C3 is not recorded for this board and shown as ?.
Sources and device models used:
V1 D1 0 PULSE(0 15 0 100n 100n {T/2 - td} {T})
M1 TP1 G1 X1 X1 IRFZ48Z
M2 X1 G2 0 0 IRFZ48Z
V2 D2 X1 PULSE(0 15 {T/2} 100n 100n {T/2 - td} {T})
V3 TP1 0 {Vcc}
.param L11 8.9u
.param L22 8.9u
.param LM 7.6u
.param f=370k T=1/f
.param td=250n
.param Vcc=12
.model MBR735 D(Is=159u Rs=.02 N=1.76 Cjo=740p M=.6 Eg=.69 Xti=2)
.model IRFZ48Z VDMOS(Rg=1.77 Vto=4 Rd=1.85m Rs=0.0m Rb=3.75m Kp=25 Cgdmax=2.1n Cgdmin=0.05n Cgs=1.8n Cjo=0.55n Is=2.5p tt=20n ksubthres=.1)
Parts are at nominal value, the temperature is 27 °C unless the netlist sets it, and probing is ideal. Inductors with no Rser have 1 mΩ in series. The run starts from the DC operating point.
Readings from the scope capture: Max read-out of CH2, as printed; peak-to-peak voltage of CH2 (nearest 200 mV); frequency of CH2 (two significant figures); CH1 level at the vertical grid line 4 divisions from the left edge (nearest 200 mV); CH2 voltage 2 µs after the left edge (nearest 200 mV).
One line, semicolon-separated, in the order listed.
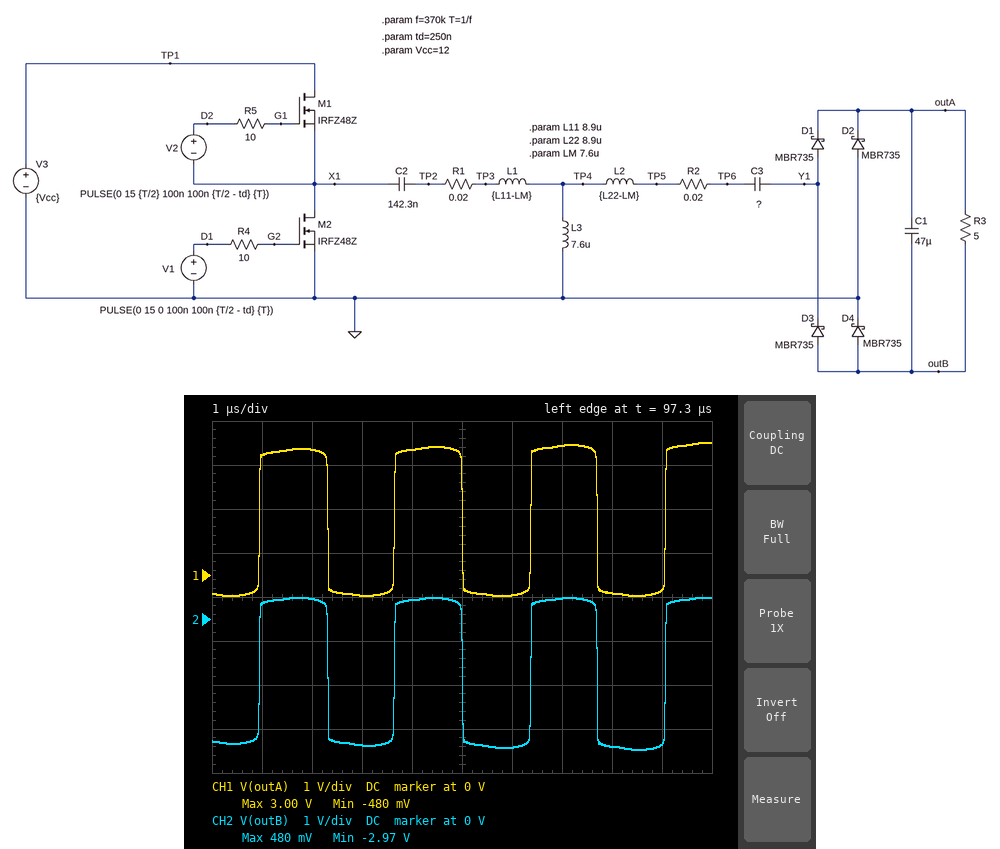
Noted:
480 mV; 3.4 V; 370 kHz; 2.8 V; 400 mV
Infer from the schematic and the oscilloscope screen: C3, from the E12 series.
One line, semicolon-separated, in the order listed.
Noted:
68 nF
